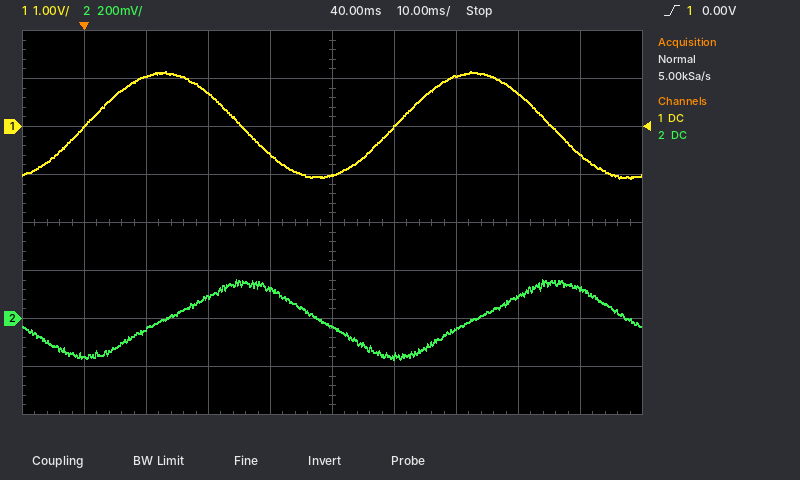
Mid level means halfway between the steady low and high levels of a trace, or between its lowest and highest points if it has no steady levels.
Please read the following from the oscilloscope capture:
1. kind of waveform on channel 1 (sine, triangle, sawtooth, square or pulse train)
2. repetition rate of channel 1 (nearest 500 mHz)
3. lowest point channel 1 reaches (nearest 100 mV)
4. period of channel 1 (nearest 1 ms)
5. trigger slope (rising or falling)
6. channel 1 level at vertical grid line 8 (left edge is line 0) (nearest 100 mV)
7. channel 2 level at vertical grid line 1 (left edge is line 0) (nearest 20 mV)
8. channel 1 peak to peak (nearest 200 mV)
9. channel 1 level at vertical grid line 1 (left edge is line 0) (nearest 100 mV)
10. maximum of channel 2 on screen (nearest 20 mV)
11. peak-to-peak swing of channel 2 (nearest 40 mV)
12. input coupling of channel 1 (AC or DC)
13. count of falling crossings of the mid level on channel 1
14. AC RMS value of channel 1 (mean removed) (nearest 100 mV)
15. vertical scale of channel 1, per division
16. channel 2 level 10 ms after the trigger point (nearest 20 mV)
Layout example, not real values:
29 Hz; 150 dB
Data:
sine; 20.0 Hz; -1.1 V; 50 ms; rising; 700 mV; -160 mV; 2.2 V; 0.0 V; 160 mV; 320 mV; DC; 2; 800 mV; 1 V; -40 mV
